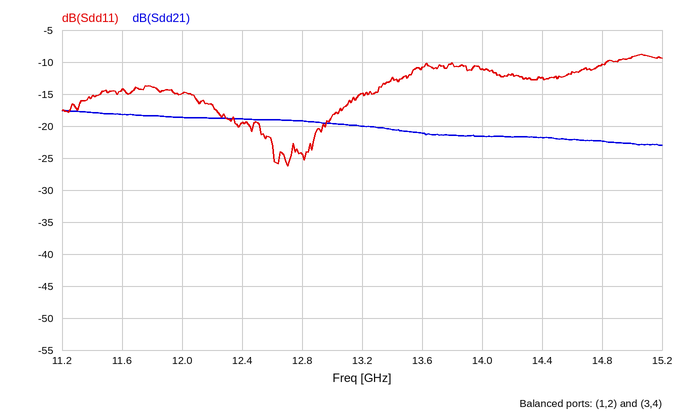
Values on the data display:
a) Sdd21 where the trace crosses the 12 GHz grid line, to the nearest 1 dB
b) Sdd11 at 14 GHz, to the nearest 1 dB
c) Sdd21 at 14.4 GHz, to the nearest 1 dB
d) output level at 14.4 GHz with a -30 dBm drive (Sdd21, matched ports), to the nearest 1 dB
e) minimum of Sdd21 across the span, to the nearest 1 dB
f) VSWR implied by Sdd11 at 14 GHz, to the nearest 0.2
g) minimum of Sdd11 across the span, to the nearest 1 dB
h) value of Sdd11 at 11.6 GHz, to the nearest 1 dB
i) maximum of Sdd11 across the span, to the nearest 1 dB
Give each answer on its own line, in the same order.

-19 dB
-11 dB
-22 dB
-52 dBm
-23 dB
1.8
-26 dB
-14 dB
-9 dB
